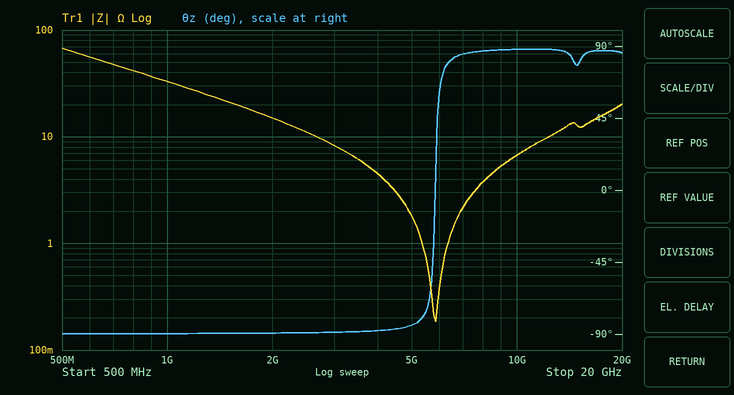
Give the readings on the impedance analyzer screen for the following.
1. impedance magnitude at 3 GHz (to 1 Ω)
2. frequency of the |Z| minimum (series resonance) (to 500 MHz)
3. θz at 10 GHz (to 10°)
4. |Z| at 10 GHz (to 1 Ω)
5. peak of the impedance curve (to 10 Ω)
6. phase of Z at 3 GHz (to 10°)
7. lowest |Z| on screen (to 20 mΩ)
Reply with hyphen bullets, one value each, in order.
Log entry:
- 8 Ω
- 6.0 GHz
- 90°
- 7 Ω
- 70 Ω
- -90°
- 180 mΩ
